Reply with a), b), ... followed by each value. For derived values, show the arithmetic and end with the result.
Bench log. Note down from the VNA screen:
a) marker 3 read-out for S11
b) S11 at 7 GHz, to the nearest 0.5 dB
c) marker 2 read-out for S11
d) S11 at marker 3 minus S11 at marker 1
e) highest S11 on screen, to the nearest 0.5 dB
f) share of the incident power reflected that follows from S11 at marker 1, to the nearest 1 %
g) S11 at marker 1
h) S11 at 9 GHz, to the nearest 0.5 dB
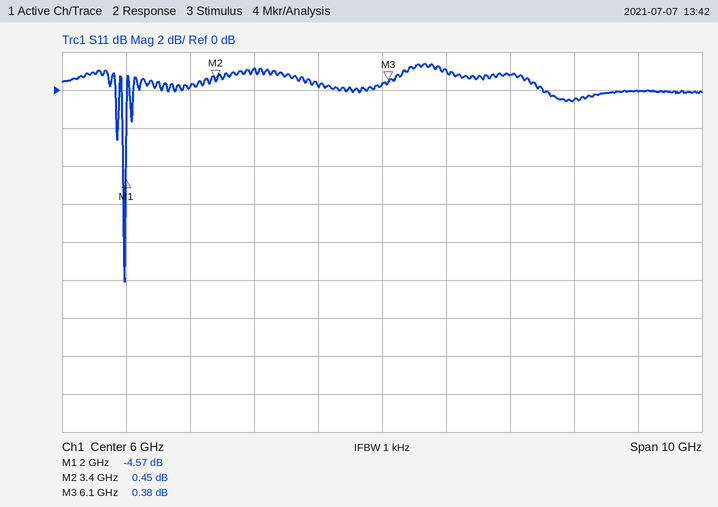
a) 0.38 dB
b) 1.0 dB
c) 0.45 dB
d) 0.38 − (-4.57) = 4.95 dB
e) 1.5 dB
f) 10^(-4.57/10) ≈ 35 %
g) -4.57 dB
h) -0.5 dB
